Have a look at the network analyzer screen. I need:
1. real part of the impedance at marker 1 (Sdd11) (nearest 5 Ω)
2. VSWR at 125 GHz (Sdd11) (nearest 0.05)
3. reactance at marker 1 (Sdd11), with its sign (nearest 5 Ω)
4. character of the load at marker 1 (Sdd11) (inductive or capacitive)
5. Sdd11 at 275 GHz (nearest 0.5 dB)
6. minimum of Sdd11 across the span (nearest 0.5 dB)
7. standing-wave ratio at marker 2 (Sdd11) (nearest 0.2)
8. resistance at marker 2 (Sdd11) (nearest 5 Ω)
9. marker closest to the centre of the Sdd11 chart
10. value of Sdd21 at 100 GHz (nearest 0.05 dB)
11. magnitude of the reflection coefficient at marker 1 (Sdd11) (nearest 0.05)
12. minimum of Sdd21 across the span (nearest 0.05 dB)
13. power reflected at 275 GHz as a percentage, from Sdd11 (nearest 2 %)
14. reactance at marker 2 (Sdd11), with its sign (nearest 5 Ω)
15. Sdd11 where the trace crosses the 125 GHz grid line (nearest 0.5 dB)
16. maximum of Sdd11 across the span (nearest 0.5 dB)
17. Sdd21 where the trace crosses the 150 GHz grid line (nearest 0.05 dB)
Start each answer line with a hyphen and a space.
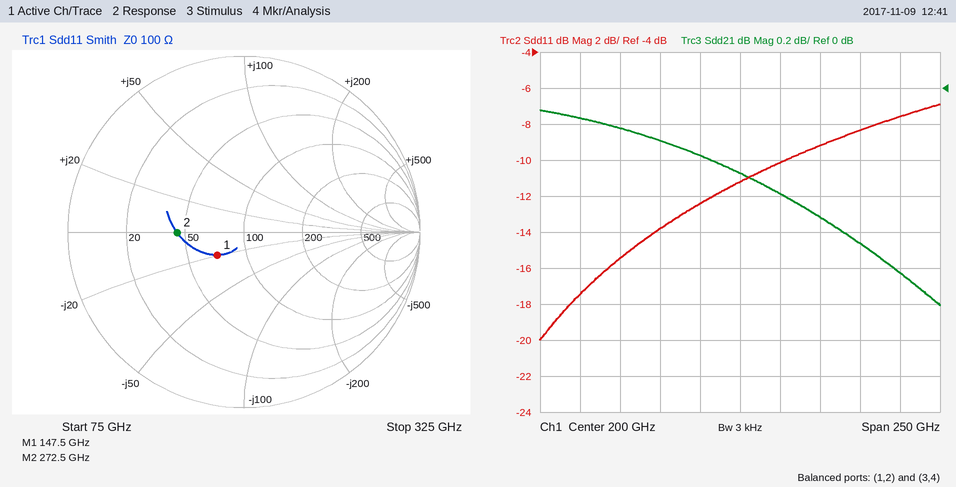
- 70 Ω
- 1.40
- -20 Ω
- capacitive
- -8.5 dB
- -20.0 dB
- 2.2
- 45 Ω
- marker 1
- -0.15 dB
- 0.20
- -1.20 dB
- 14 %
- 0 Ω
- -15.5 dB
- -7.0 dB
- -0.30 dB
